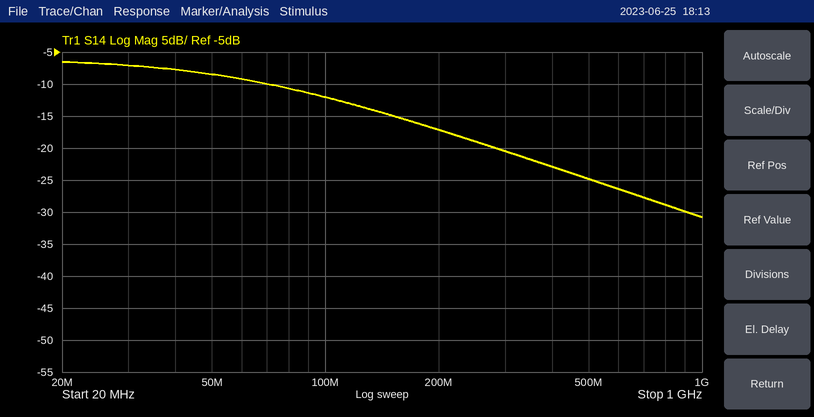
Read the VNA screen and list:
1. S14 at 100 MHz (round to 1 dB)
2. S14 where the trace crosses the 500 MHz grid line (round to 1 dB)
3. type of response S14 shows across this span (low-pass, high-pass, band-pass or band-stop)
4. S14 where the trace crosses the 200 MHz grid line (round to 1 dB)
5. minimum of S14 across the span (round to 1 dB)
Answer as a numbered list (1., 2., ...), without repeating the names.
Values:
1. -12 dB
2. -25 dB
3. low-pass
4. -17 dB
5. -31 dB
